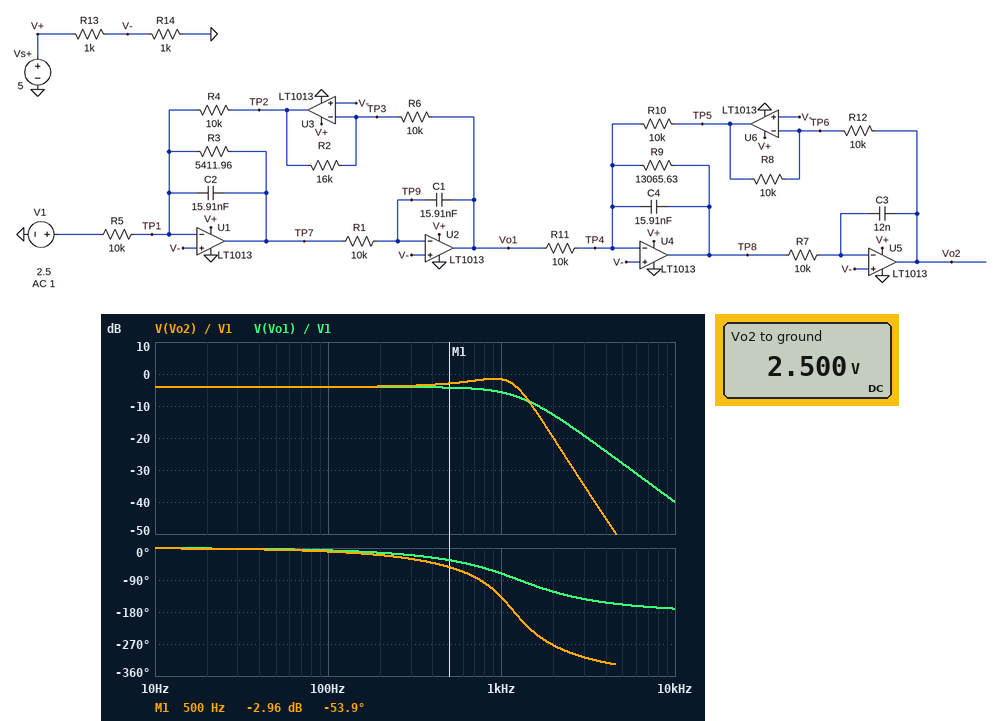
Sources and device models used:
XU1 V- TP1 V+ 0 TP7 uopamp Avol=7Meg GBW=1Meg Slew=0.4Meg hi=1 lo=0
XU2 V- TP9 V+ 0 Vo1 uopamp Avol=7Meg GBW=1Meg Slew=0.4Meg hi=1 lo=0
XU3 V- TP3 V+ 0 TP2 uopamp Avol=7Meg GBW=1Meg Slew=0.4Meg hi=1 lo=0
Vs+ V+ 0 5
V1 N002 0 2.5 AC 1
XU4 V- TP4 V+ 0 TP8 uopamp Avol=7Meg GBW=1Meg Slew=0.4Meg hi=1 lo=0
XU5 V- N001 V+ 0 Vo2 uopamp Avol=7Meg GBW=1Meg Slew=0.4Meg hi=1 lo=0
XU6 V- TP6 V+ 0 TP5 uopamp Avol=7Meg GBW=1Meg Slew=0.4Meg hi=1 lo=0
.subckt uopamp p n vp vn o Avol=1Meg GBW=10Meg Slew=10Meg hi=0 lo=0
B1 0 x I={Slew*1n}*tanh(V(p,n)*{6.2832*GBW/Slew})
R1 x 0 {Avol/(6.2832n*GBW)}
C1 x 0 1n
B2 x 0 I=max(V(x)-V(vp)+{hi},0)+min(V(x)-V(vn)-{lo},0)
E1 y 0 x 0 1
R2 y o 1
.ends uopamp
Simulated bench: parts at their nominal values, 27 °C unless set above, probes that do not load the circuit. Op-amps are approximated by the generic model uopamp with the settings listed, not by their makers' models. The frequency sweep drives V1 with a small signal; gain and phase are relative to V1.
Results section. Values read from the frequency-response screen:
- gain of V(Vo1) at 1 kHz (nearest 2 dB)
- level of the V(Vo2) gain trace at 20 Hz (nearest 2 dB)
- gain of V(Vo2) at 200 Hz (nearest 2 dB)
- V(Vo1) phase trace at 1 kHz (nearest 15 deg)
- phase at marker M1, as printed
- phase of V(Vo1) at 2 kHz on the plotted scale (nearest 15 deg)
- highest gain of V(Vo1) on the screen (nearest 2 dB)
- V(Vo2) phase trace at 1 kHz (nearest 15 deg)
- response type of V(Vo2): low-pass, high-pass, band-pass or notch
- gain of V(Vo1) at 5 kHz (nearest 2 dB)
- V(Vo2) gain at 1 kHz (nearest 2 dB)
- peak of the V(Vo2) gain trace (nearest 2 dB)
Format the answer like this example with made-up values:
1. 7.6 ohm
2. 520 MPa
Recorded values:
1. -6 dB
2. -4 dB
3. -4 dB
4. -75 deg
5. -53.9 deg
6. -120 deg
7. -4 dB
8. -135 deg
9. low-pass
10. -28 dB
11. -2 dB
12. -2 dB
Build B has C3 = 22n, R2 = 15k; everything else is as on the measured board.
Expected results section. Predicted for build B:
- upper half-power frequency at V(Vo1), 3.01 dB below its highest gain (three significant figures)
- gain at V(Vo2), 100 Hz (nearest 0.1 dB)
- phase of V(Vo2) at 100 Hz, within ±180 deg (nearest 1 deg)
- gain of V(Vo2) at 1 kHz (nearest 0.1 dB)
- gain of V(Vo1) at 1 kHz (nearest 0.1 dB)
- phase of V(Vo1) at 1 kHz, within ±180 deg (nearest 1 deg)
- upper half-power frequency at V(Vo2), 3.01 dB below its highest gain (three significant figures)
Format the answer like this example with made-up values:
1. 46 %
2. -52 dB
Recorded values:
1. 1.15 kHz
2. -3.5 dB
3. -13 deg
4. -6.6 dB
5. -5.6 dB
6. -75 deg
7. 926 Hz
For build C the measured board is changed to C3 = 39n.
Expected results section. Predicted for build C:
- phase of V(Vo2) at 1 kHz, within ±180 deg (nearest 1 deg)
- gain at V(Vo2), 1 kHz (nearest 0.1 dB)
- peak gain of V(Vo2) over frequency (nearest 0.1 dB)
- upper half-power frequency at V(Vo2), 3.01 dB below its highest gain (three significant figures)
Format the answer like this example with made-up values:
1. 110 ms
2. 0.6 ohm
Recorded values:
1. 160 deg
2. -13.2 dB
3. -3.8 dB
4. 684 Hz
